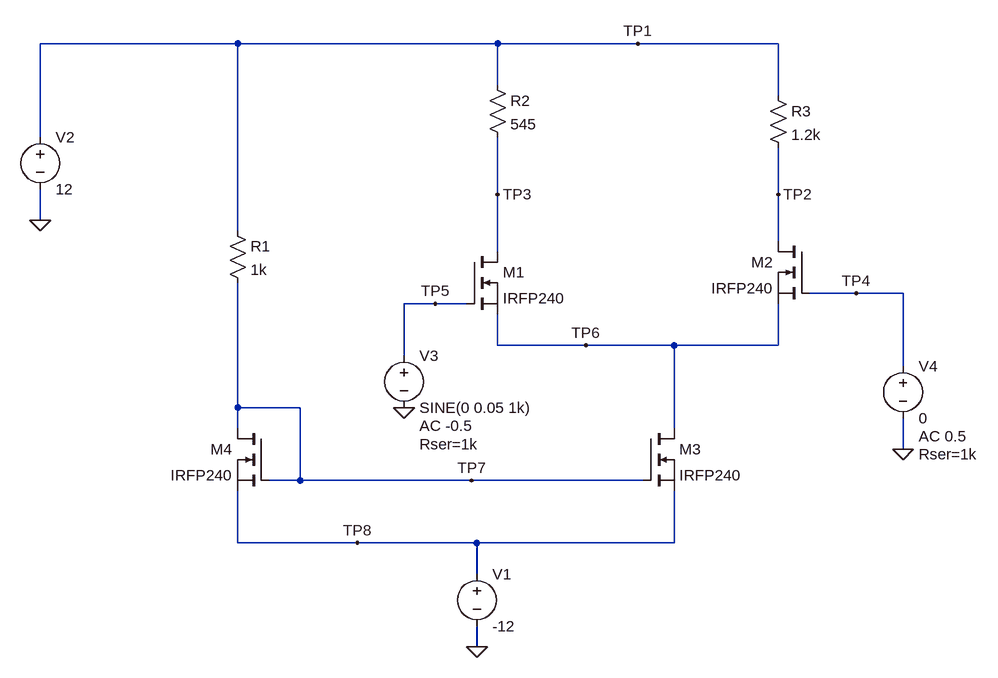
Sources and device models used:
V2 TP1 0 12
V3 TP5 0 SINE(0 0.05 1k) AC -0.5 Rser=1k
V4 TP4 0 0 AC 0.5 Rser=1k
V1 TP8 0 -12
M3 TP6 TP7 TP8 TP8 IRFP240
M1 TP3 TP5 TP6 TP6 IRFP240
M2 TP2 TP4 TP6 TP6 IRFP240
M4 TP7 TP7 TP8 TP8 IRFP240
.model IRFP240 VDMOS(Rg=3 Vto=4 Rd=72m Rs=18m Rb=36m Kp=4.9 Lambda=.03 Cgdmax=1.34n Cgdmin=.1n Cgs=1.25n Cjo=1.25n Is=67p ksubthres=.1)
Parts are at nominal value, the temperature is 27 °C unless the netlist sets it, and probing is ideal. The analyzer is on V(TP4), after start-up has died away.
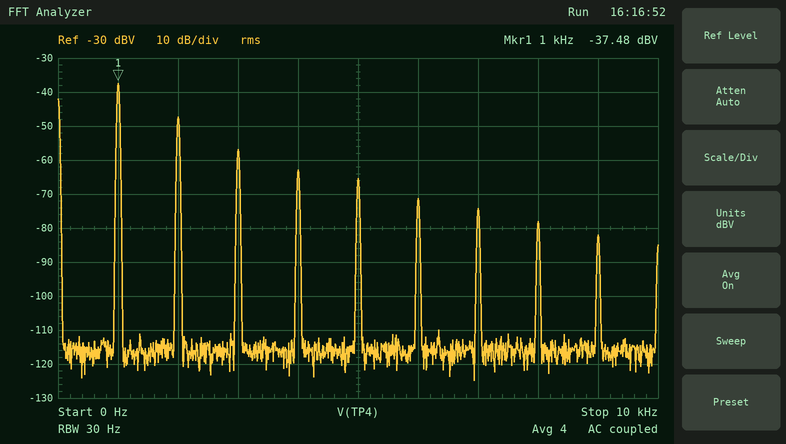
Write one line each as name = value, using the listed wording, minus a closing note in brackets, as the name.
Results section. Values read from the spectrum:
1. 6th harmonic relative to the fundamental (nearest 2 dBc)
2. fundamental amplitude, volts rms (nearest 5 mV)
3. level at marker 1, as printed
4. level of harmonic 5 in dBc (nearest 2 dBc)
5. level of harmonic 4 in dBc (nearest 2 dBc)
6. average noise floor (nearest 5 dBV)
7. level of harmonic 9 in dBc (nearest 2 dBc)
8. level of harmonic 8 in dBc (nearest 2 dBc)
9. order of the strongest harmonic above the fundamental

6th harmonic relative to the fundamental = -34 dBc
fundamental amplitude, volts rms = 15 mV
level at marker 1, as printed = -37.48 dBV
level of harmonic 5 in dBc = -28 dBc
level of harmonic 4 in dBc = -26 dBc
average noise floor = -115 dBV
level of harmonic 9 in dBc = -44 dBc
level of harmonic 8 in dBc = -40 dBc
order of the strongest harmonic above the fundamental = 2
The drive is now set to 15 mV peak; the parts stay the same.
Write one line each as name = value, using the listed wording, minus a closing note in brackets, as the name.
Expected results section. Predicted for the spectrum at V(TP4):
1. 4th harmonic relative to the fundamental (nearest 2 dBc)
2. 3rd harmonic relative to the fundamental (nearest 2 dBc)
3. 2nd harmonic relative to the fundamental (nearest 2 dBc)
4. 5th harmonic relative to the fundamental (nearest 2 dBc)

4th harmonic relative to the fundamental = -42 dBc
3rd harmonic relative to the fundamental = -30 dBc
2nd harmonic relative to the fundamental = -16 dBc
5th harmonic relative to the fundamental = -50 dBc
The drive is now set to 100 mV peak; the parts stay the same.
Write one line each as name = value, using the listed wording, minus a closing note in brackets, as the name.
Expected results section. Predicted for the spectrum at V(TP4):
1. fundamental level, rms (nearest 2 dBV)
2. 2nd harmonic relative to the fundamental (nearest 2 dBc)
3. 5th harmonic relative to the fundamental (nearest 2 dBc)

fundamental level, rms = -34 dBV
2nd harmonic relative to the fundamental = -16 dBc
5th harmonic relative to the fundamental = -20 dBc
